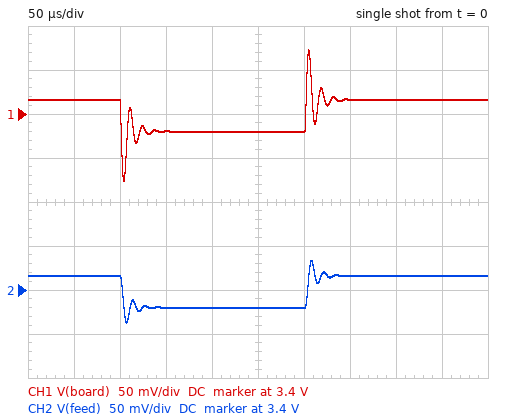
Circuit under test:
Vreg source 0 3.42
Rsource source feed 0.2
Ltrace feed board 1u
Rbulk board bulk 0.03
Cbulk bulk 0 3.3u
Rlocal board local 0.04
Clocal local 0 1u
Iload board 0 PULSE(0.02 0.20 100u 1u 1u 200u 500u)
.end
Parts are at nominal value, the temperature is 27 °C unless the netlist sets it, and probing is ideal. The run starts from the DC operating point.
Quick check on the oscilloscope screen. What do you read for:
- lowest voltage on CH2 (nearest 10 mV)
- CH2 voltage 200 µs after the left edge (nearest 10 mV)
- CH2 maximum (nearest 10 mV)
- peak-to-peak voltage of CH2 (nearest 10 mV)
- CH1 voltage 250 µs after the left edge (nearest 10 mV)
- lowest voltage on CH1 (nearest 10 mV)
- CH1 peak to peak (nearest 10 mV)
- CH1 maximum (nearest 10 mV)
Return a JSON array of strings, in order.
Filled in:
["3.36 V", "3.38 V", "3.43 V", "70 mV", "3.38 V", "3.32 V", "150 mV", "3.47 V"]
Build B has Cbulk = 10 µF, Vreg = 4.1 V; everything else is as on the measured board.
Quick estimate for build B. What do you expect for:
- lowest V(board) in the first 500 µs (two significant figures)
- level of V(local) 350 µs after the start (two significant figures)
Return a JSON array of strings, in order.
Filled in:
["4.0 V", "4.1 V"]
